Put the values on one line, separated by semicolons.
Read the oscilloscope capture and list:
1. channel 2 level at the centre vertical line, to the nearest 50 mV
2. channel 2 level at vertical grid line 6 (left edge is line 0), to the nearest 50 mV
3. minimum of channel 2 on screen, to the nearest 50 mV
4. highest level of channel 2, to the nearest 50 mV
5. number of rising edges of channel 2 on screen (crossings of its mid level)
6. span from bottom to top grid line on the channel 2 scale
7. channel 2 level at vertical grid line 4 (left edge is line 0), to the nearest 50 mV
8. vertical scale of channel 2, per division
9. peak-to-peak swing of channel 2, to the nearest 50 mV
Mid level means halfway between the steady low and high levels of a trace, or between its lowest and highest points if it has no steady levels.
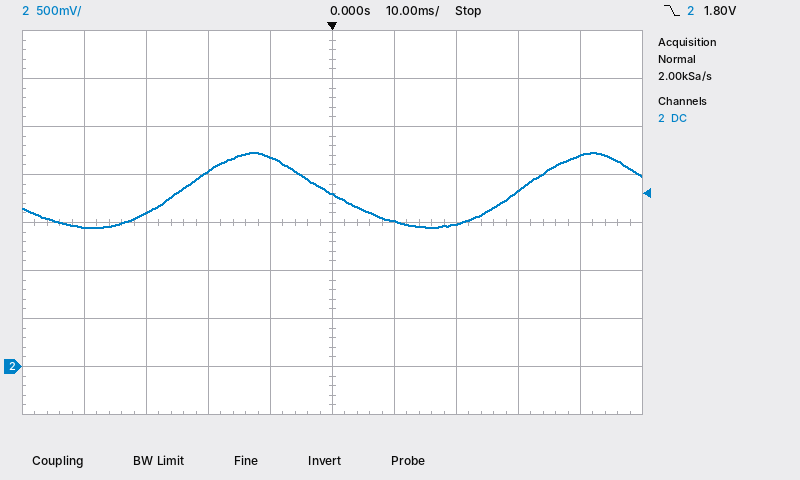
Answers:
1.80 V; 1.50 V; 1.45 V; 2.25 V; 2; 4 V; 2.20 V; 500 mV; 800 mV
